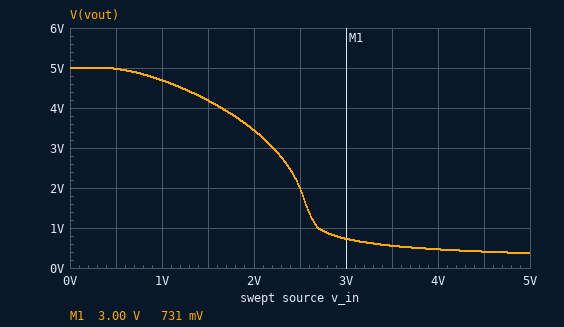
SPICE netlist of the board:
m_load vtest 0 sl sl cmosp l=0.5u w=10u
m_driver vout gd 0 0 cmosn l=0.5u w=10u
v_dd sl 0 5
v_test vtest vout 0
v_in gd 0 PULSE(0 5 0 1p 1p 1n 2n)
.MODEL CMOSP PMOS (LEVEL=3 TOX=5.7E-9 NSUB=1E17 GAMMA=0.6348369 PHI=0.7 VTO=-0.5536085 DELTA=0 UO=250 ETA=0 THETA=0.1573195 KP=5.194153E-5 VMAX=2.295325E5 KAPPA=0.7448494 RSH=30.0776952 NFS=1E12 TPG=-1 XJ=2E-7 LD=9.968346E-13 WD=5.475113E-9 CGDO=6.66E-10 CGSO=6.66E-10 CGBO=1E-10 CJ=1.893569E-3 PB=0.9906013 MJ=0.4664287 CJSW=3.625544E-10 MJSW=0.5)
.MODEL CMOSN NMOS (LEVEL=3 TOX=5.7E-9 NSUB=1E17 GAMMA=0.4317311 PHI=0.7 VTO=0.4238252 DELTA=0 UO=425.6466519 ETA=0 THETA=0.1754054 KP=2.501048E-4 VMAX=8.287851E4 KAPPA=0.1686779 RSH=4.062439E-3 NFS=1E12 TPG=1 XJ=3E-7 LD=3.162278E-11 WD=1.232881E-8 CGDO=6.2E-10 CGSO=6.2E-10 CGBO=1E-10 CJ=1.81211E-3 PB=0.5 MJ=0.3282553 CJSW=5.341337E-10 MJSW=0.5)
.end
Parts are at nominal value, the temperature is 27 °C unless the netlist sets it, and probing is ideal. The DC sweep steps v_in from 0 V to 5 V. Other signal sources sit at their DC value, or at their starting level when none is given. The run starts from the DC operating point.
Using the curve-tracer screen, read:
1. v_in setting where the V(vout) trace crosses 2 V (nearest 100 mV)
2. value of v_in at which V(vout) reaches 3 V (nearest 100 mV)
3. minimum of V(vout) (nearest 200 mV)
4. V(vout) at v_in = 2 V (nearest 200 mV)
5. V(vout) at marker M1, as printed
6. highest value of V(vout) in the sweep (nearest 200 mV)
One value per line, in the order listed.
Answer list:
2.5 V
2.2 V
400 mV
3.4 V
731 mV
5.0 V
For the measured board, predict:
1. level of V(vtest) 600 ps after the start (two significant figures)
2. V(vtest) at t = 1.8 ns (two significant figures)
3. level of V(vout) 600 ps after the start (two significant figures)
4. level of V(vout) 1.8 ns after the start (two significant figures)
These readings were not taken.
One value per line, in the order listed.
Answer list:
370 mV
5.0 V
370 mV
5.0 V
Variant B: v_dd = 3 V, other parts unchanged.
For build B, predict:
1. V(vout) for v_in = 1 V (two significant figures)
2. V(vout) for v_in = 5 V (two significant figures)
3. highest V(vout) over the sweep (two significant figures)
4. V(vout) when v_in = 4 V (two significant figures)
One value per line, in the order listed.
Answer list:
2.6 V
130 mV
3.0 V
160 mV
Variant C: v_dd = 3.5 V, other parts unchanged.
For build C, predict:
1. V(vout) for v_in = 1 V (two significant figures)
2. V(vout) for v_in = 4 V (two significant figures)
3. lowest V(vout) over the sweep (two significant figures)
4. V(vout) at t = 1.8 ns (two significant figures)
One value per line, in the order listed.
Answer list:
3.1 V
220 mV
180 mV
3.5 V
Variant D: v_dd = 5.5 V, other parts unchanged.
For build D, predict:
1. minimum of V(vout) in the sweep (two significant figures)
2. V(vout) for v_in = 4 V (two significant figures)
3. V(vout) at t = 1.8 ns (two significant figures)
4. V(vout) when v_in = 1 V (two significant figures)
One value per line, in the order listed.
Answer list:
450 mV
580 mV
5.5 V
5.2 V
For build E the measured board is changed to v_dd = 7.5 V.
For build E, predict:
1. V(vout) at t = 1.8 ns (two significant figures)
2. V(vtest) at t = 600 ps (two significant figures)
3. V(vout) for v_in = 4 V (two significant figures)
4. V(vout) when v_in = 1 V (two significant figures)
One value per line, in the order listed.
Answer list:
7.5 V
910 mV
1.8 V
7.2 V
